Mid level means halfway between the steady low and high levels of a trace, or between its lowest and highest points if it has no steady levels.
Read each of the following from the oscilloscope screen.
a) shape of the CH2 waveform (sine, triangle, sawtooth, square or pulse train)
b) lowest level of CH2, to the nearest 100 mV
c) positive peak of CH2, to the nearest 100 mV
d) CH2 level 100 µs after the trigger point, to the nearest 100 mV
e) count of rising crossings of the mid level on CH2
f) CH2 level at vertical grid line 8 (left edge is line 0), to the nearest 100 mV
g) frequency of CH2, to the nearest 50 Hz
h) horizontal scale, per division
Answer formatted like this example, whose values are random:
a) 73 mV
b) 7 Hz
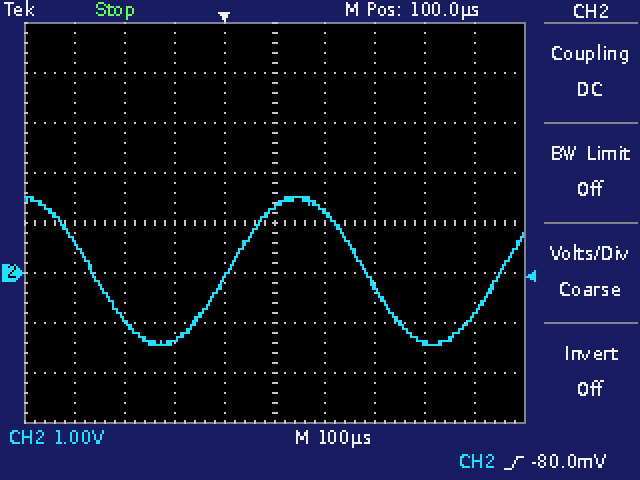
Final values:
a) sine
b) -1.4 V
c) 1.5 V
d) 1.3 V
e) 2
f) -1.4 V
g) 1.85 kHz
h) 100 µs
